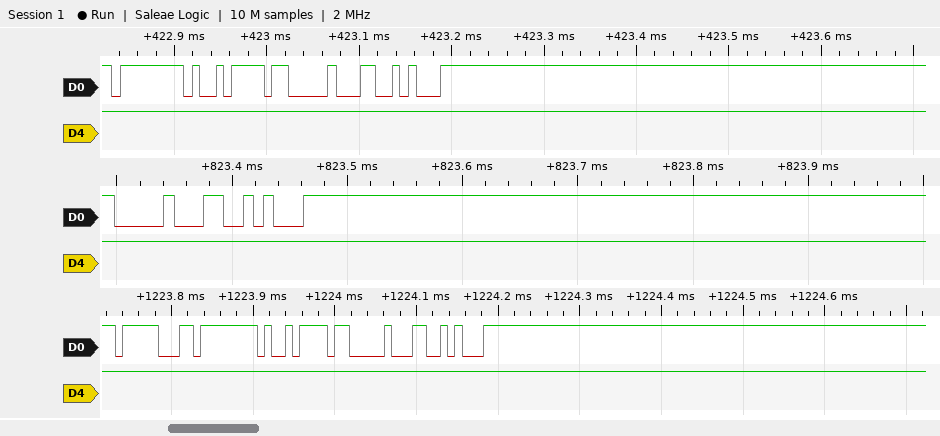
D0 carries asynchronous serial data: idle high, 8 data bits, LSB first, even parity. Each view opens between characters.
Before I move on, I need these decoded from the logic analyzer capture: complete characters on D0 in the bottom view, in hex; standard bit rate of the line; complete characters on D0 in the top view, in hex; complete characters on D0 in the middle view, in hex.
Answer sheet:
1F, FF, 7A, 10, 8A
115200 baud
FF, 7A, 10, 8A
10, 8A
